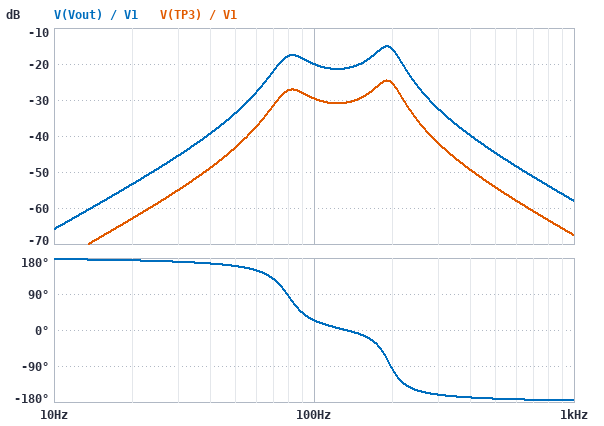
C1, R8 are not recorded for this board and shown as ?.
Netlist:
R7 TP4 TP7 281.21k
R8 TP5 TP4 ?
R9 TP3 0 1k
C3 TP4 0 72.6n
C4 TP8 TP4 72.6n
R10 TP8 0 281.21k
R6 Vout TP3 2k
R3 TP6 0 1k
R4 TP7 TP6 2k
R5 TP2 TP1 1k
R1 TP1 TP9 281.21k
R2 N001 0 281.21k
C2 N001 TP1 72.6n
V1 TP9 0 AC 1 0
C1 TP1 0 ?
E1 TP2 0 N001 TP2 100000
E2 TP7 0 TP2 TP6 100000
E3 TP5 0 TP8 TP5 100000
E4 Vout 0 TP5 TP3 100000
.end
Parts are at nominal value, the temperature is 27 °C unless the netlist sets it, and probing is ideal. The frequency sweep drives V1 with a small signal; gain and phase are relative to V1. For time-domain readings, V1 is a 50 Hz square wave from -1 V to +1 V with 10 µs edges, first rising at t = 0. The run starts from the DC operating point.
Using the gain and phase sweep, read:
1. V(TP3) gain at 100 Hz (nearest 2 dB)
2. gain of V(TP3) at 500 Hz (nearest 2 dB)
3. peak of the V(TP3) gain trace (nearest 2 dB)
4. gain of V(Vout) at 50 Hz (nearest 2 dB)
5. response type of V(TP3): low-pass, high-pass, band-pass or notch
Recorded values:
-30 dB
-54 dB
-24 dB
-34 dB
band-pass
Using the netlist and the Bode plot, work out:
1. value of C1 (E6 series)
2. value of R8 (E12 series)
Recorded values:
33 nF
2.7 kΩ
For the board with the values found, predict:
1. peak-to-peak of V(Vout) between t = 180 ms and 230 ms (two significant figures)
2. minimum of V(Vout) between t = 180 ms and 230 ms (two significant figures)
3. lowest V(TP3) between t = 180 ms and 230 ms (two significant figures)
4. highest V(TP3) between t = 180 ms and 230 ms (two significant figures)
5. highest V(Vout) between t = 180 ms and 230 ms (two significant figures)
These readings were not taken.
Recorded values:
150 mV
-76 mV
-25 mV
25 mV
76 mV
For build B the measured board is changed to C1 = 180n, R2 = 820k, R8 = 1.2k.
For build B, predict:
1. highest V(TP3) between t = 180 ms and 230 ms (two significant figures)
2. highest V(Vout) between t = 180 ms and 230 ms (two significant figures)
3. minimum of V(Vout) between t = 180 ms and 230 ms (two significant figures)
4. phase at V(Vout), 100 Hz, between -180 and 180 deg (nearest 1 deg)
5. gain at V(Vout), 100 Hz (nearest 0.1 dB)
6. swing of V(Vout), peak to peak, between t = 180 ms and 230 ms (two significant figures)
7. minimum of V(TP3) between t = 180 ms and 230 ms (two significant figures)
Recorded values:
50 mV
150 mV
-150 mV
-23 deg
-24.6 dB
300 mV
-50 mV
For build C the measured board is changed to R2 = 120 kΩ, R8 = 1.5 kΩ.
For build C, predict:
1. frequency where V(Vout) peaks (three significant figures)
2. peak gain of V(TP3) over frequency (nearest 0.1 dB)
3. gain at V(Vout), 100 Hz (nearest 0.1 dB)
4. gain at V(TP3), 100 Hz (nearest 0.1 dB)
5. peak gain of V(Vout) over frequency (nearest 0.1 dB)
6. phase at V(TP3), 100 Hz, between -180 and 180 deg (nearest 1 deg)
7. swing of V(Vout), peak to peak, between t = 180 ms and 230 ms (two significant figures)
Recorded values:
109 Hz
-32.4 dB
-25.1 dB
-34.7 dB
-22.9 dB
116 deg
61 mV
